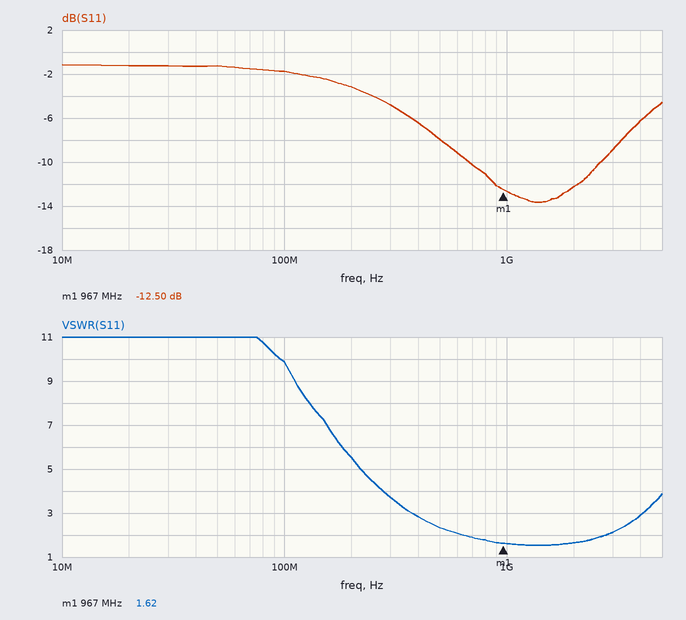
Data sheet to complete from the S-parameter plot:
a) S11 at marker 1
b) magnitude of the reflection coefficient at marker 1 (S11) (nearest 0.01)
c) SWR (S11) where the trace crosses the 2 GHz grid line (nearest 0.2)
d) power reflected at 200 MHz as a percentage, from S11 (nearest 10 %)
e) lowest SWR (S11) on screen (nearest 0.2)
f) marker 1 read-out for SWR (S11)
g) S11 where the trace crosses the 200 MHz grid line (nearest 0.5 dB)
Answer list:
-12.50 dB
0.24
1.6
50 %
1.6
1.62
-3.0 dB
